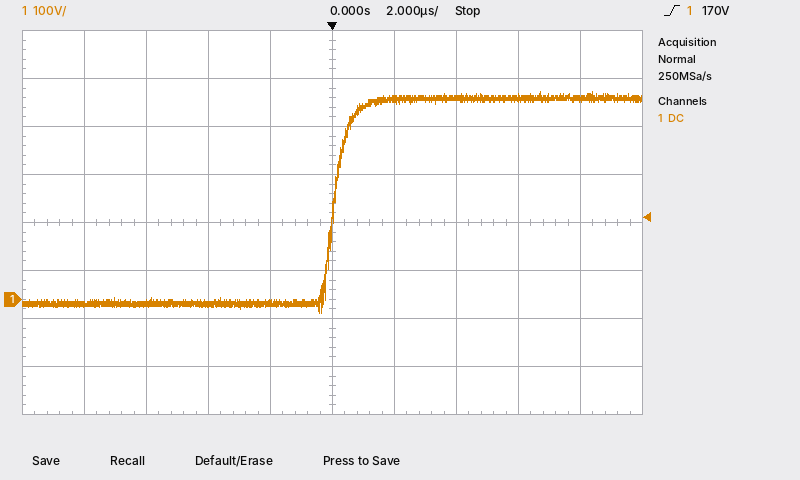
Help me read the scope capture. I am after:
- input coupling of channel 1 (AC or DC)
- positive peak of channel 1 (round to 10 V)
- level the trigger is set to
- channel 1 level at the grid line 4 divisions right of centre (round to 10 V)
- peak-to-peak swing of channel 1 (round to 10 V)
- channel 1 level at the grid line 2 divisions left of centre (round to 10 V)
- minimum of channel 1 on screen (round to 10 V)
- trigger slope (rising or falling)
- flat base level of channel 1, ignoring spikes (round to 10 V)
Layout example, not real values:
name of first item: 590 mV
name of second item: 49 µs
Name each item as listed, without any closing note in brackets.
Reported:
input coupling of channel 1: DC
positive peak of channel 1: 430 V
level the trigger is set to: 170 V
channel 1 level at the grid line 4 divisions right of centre: 420 V
peak-to-peak swing of channel 1: 460 V
channel 1 level at the grid line 2 divisions left of centre: -10 V
minimum of channel 1 on screen: -30 V
trigger slope: rising
flat base level of channel 1, ignoring spikes: -10 V
